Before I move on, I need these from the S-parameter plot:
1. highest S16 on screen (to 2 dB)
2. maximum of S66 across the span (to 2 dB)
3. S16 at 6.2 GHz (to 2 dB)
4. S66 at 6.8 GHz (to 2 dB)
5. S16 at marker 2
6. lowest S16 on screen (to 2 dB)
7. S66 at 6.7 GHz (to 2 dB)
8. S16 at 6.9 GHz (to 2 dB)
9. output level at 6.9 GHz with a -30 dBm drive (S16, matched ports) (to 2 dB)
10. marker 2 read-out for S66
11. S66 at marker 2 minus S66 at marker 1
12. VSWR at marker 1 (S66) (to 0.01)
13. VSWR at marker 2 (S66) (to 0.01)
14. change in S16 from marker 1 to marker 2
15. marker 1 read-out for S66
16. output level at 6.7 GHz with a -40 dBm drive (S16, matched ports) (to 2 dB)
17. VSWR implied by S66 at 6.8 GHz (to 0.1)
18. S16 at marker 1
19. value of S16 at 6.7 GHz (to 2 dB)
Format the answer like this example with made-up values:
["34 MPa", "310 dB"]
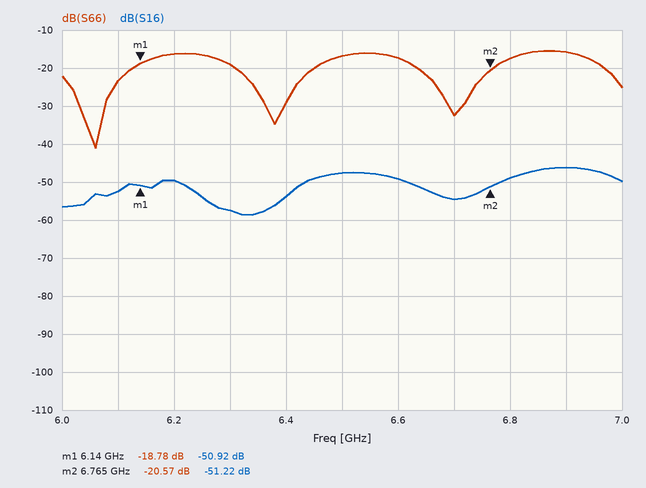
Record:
["-46 dB", "-16 dB", "-50 dB", "-18 dB", "-51.22 dB", "-58 dB", "-32 dB", "-46 dB", "-76 dBm", "-20.57 dB", "-1.79 dB", "1.26", "1.21", "-0.30 dB", "-18.78 dB", "-94 dBm", "1.3", "-50.92 dB", "-54 dB"]
